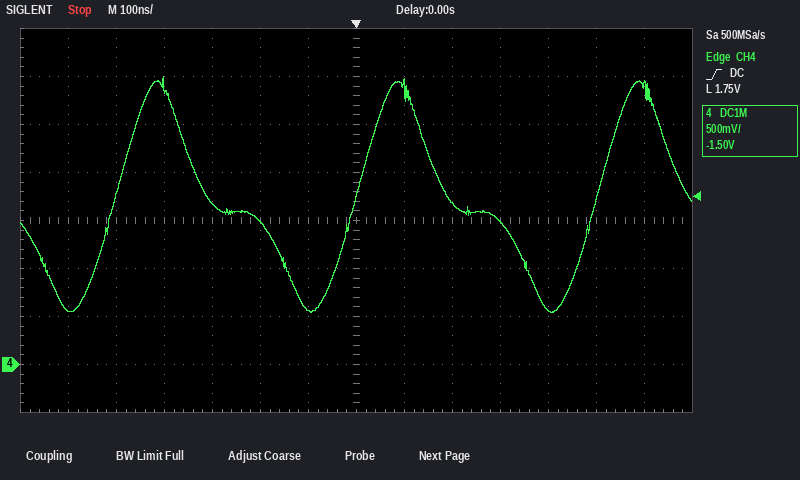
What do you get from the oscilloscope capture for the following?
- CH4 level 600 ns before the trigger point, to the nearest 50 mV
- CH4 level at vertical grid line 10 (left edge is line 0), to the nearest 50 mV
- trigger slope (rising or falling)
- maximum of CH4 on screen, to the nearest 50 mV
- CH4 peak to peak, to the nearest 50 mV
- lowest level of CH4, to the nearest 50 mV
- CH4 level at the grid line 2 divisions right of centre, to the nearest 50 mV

550 mV
1.50 V
rising
3.00 V
2.45 V
550 mV
1.70 V
